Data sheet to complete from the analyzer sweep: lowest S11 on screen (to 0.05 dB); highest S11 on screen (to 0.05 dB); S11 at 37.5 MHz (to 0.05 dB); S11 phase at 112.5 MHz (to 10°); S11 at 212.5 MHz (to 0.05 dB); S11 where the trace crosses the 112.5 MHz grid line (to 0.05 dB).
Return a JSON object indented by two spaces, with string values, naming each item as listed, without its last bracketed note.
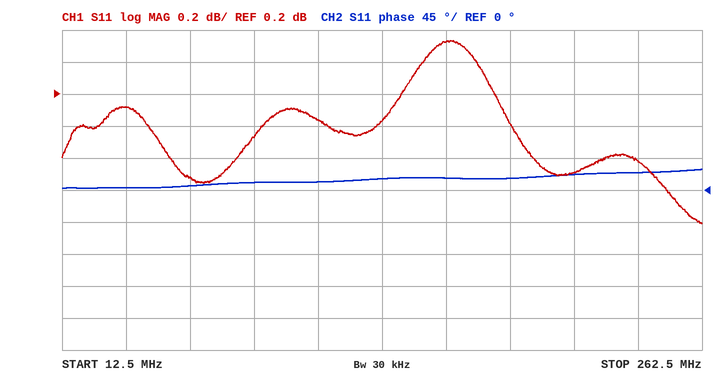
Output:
{
  "lowest S11 on screen": "-0.60 dB",
  "highest S11 on screen": "0.55 dB",
  "S11 at 37.5 MHz": "0.10 dB",
  "S11 phase at 112.5 MHz": "10°",
  "S11 at 212.5 MHz": "-0.30 dB",
  "S11 where the trace crosses the 112.5 MHz grid line": "0.05 dB"
}
